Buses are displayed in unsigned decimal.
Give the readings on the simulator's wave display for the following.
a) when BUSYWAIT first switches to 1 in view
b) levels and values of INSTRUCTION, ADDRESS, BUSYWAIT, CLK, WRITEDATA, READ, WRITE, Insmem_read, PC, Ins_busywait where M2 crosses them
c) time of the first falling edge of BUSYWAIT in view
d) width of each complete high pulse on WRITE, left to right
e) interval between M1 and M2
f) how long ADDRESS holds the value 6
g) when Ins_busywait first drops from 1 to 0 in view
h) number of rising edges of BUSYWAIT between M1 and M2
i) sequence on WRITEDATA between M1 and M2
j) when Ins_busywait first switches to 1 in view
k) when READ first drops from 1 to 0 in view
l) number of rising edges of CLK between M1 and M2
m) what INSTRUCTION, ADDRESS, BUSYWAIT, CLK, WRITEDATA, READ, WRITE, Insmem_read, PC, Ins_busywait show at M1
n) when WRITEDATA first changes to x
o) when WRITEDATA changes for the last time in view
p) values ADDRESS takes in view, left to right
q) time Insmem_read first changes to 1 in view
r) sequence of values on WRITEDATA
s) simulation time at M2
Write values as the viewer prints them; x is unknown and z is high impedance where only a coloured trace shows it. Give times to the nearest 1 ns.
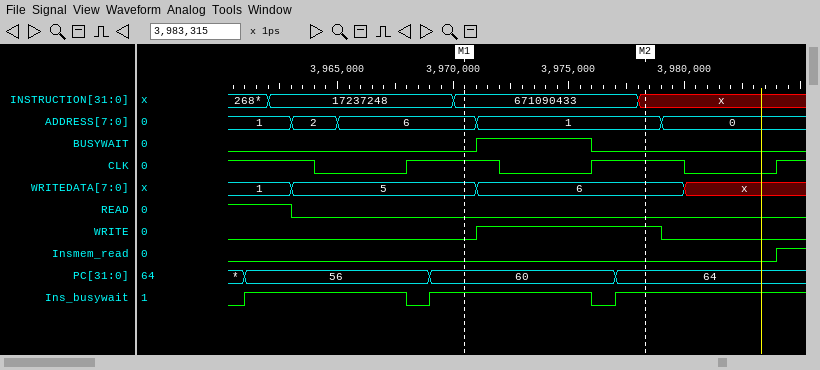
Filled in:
3971 ns
INSTRUCTION=x, ADDRESS=1, BUSYWAIT=0, CLK=1, WRITEDATA=6, READ=0, WRITE=1, Insmem_read=0, PC=64, Ins_busywait=1
3976 ns
8 ns
8 ns
6 ns
3968 ns
1
5, 6
3961 ns
3963 ns
1
INSTRUCTION=671090433, ADDRESS=6, BUSYWAIT=0, CLK=1, WRITEDATA=5, READ=0, WRITE=0, Insmem_read=0, PC=60, Ins_busywait=1
3980 ns
3980 ns
1, 2, 6, 1, 0
3984 ns
1, 5, 6, x
3978 ns
